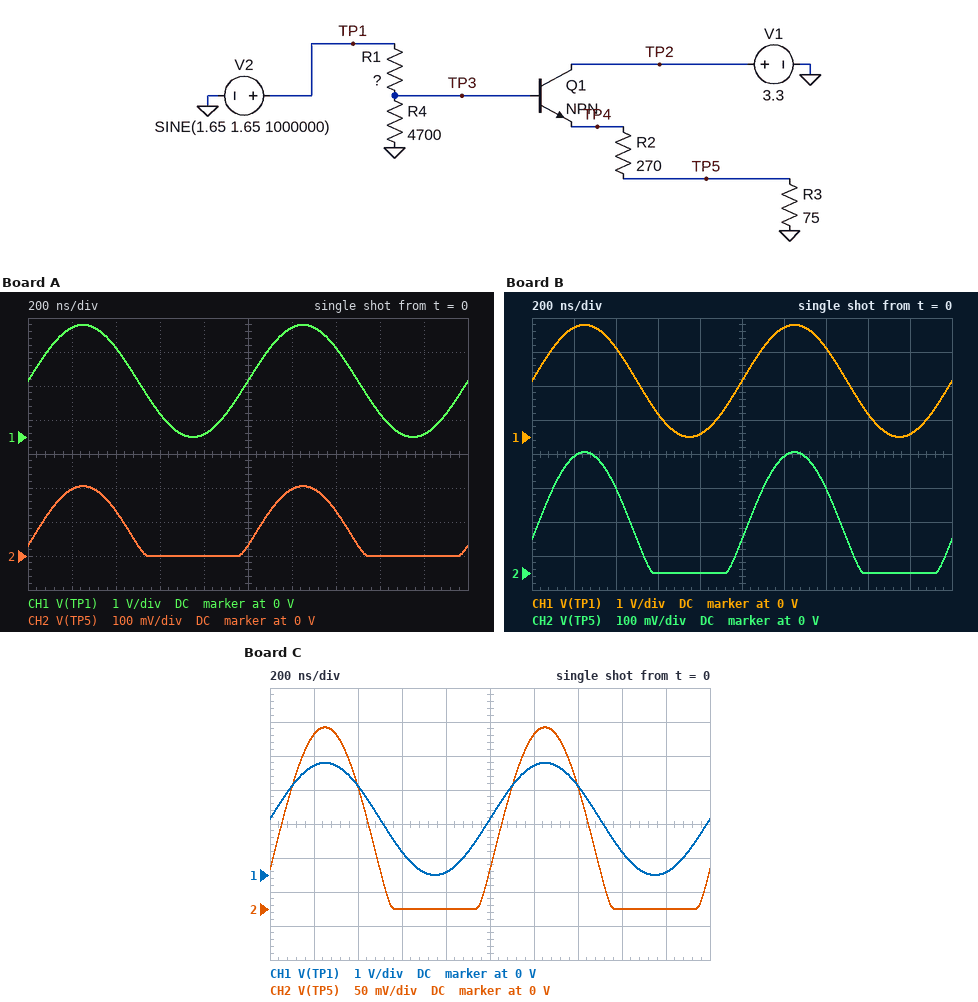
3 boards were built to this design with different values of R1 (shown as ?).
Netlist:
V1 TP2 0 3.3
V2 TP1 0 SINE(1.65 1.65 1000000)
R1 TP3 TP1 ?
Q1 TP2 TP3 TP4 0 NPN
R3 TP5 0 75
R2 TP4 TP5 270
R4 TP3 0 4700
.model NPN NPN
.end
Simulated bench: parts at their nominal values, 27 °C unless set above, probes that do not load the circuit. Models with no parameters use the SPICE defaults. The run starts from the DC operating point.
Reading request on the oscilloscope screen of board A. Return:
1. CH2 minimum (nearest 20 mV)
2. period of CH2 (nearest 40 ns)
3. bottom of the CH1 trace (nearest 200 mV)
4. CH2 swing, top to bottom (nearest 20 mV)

0 V
1.00 µs
0 V
200 mV
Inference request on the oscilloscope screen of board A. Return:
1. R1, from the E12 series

3.9 kΩ
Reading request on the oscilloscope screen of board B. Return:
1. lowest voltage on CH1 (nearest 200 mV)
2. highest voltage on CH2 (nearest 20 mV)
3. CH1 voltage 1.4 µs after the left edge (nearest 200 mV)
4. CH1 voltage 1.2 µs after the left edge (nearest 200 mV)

0 V
360 mV
2.6 V
3.2 V
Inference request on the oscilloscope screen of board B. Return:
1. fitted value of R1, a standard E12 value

1.5 kΩ
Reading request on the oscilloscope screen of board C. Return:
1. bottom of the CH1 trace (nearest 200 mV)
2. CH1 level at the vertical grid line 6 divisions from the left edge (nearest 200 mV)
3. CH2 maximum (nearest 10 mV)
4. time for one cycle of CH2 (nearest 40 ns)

0 V
3.2 V
270 mV
1.00 µs
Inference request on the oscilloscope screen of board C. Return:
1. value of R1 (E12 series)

2.7 kΩ
